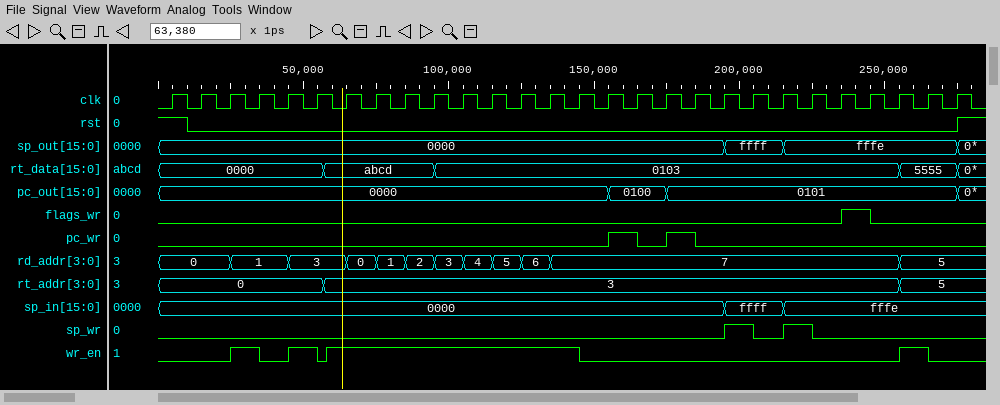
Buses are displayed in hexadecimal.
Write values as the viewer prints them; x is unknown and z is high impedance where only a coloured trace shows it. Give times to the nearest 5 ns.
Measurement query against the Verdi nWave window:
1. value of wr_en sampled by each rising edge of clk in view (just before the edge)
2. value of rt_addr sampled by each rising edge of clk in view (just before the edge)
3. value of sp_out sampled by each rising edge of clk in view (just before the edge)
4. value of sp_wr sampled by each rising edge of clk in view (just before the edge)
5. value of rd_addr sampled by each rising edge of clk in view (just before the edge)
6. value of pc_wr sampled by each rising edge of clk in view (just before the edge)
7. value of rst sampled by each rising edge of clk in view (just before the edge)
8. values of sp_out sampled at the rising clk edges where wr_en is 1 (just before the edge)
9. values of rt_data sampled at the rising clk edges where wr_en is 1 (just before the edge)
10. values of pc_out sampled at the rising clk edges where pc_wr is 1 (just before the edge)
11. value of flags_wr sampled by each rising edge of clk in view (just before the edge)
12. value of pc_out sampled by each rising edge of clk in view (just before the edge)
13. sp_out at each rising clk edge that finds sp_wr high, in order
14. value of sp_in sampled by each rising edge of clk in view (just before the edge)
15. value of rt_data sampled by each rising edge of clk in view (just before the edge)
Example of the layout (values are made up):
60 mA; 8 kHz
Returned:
0 0 0 1 0 1 1 1 1 1 1 1 1 1 1 0 0 0 0 0 0 0 0 0 0 0 1 0; 0, 0, 0, 0, 0, 0, 3, 3, 3, 3, 3, 3, 3, 3, 3, 3, 3, 3, 3, 3, 3, 3, 3, 3, 3, 3, 5, 5; 0000, 0000, 0000, 0000, 0000, 0000, 0000, 0000, 0000, 0000, 0000, 0000, 0000, 0000, 0000, 0000, 0000, 0000, 0000, 0000, ffff, ffff, fffe, fffe, fffe, fffe, fffe, fffe; 0 0 0 0 0 0 0 0 0 0 0 0 0 0 0 0 0 0 0 0 1 0 1 0 0 0 0 0; 0, 0, 0, 1, 1, 3, 3, 0, 1, 2, 3, 4, 5, 6, 7, 7, 7, 7, 7, 7, 7, 7, 7, 7, 7, 7, 5, 5; 0 0 0 0 0 0 0 0 0 0 0 0 0 0 0 0 1 0 1 0 0 0 0 0 0 0 0 0; 1 0 0 0 0 0 0 0 0 0 0 0 0 0 0 0 0 0 0 0 0 0 0 0 0 0 0 0; 0000, 0000, 0000, 0000, 0000, 0000, 0000, 0000, 0000, 0000, 0000, fffe; 0000, 0000, abcd, abcd, abcd, abcd, 0103, 0103, 0103, 0103, 0103, 5555; 0100, 0101; 0 0 0 0 0 0 0 0 0 0 0 0 0 0 0 0 0 0 0 0 0 0 0 0 1 0 0 0; 0000, 0000, 0000, 0000, 0000, 0000, 0000, 0000, 0000, 0000, 0000, 0000, 0000, 0000, 0000, 0000, 0100, 0100, 0101, 0101, 0101, 0101, 0101, 0101, 0101, 0101, 0101, 0101; ffff, fffe; 0000, 0000, 0000, 0000, 0000, 0000, 0000, 0000, 0000, 0000, 0000, 0000, 0000, 0000, 0000, 0000, 0000, 0000, 0000, 0000, ffff, ffff, fffe, fffe, fffe, fffe, fffe, fffe; 0000, 0000, 0000, 0000, 0000, 0000, abcd, abcd, abcd, abcd, 0103, 0103, 0103, 0103, 0103, 0103, 0103, 0103, 0103, 0103, 0103, 0103, 0103, 0103, 0103, 0103, 5555, 5555
